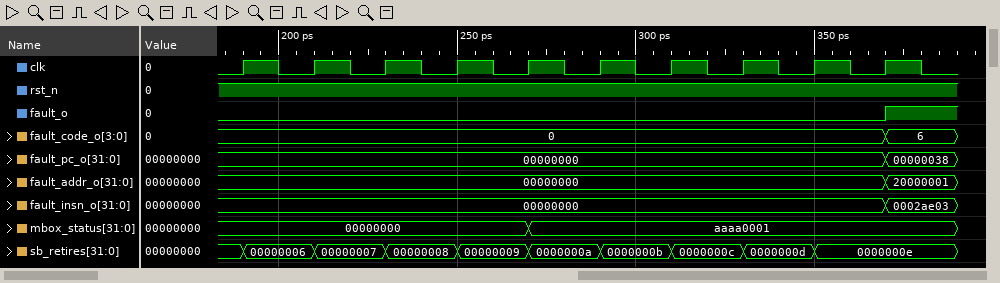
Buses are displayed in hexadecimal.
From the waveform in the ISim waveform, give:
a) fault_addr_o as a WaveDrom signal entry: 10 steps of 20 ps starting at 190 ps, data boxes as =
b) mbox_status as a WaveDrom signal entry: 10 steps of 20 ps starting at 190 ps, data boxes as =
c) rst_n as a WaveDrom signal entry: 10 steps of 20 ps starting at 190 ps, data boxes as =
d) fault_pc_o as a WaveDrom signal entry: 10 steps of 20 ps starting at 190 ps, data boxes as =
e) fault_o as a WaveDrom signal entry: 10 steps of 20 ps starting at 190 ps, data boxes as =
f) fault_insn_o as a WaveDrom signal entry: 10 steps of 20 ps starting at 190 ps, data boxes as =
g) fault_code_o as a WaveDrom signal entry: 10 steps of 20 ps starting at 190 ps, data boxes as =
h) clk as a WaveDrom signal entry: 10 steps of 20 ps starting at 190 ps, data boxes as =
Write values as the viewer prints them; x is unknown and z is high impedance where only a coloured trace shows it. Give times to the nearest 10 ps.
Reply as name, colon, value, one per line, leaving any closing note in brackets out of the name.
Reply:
fault_addr_o as a WaveDrom signal entry: 10 steps of 20 ps starting at 190 ps, data boxes as =: {name: 'fault_addr_o', wave: '=........=', data: '00000000 20000001'}
mbox_status as a WaveDrom signal entry: 10 steps of 20 ps starting at 190 ps, data boxes as =: {name: 'mbox_status', wave: '=...=.....', data: '00000000 aaaa0001'}
rst_n as a WaveDrom signal entry: 10 steps of 20 ps starting at 190 ps, data boxes as =: {name: 'rst_n', wave: '1.........'}
fault_pc_o as a WaveDrom signal entry: 10 steps of 20 ps starting at 190 ps, data boxes as =: {name: 'fault_pc_o', wave: '=........=', data: '00000000 00000038'}
fault_o as a WaveDrom signal entry: 10 steps of 20 ps starting at 190 ps, data boxes as =: {name: 'fault_o', wave: '0........1'}
fault_insn_o as a WaveDrom signal entry: 10 steps of 20 ps starting at 190 ps, data boxes as =: {name: 'fault_insn_o', wave: '=........=', data: '00000000 0002ae03'}
fault_code_o as a WaveDrom signal entry: 10 steps of 20 ps starting at 190 ps, data boxes as =: {name: 'fault_code_o', wave: '=........=', data: '0 6'}
clk as a WaveDrom signal entry: 10 steps of 20 ps starting at 190 ps, data boxes as =: {name: 'clk', wave: 'p.........'}
